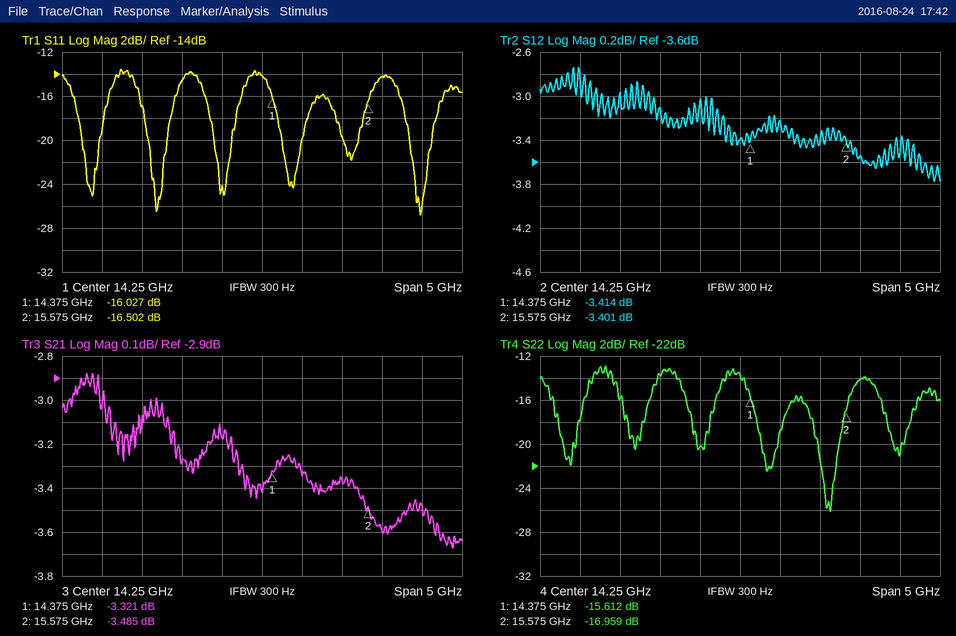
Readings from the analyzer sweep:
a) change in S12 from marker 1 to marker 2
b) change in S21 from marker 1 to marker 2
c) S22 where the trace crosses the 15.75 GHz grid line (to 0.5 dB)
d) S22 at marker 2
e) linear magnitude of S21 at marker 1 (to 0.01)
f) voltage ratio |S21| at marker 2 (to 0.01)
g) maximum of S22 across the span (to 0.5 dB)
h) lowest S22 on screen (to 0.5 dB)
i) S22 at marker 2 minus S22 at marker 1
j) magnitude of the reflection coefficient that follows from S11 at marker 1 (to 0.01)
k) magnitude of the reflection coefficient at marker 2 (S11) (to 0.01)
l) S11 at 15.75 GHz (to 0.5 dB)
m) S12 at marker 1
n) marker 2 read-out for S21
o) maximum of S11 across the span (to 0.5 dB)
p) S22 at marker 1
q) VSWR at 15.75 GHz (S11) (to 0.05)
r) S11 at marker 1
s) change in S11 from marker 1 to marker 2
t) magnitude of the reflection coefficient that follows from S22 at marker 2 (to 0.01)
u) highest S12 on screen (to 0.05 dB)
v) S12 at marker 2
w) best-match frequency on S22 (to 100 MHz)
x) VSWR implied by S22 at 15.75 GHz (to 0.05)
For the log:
0.013 dB
-0.164 dB
-14.0 dB
-16.959 dB
0.68
0.67
-13.0 dB
-26.0 dB
-1.347 dB
0.16
0.15
-14.0 dB
-3.414 dB
-3.485 dB
-13.5 dB
-15.612 dB
1.50
-16.027 dB
-0.475 dB
0.14
-2.75 dB
-3.401 dB
15.4 GHz
1.50
